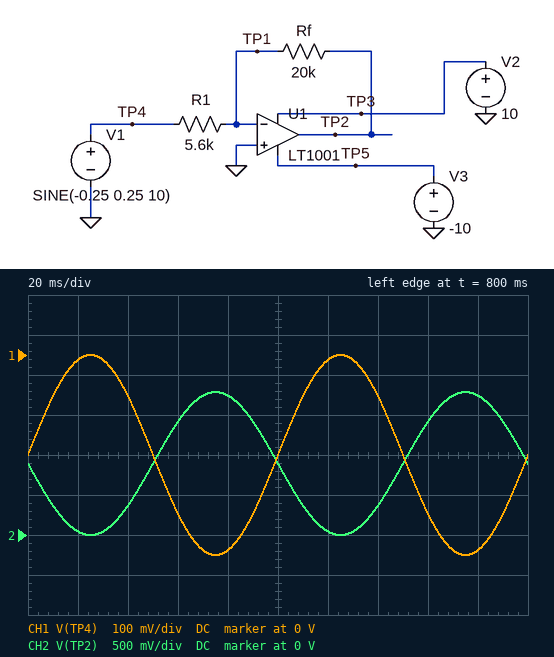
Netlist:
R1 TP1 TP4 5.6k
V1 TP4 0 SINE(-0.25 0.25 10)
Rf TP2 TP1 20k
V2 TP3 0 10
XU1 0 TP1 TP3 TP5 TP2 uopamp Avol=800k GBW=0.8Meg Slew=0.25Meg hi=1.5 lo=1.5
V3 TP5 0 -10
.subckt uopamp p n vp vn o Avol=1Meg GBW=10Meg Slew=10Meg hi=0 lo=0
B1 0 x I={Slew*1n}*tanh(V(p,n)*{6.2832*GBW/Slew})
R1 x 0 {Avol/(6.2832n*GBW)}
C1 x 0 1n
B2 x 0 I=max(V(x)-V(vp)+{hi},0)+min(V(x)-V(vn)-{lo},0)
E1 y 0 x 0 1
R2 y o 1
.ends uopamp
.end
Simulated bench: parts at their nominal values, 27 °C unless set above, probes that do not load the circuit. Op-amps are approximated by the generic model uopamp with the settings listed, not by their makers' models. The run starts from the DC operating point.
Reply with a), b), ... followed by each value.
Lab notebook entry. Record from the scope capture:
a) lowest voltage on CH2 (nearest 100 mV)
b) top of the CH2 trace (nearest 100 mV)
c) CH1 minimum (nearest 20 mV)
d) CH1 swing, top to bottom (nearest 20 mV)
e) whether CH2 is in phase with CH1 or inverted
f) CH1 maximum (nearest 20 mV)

a) 0 V
b) 1.8 V
c) -500 mV
d) 500 mV
e) inverted
f) 0 V
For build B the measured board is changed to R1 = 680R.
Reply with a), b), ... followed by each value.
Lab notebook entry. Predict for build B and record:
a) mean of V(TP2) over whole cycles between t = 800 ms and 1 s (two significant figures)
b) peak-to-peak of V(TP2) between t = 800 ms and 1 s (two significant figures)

a) 5.6 V
b) 8.5 V
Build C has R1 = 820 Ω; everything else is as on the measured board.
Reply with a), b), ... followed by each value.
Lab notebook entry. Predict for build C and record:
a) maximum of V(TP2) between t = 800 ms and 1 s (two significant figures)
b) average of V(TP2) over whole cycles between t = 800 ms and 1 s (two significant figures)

a) 8.5 V
b) 5.2 V
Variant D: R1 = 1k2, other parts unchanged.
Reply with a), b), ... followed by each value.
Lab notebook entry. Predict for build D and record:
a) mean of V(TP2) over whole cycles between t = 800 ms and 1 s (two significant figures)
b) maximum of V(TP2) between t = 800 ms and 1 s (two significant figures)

a) 4.2 V
b) 8.3 V
